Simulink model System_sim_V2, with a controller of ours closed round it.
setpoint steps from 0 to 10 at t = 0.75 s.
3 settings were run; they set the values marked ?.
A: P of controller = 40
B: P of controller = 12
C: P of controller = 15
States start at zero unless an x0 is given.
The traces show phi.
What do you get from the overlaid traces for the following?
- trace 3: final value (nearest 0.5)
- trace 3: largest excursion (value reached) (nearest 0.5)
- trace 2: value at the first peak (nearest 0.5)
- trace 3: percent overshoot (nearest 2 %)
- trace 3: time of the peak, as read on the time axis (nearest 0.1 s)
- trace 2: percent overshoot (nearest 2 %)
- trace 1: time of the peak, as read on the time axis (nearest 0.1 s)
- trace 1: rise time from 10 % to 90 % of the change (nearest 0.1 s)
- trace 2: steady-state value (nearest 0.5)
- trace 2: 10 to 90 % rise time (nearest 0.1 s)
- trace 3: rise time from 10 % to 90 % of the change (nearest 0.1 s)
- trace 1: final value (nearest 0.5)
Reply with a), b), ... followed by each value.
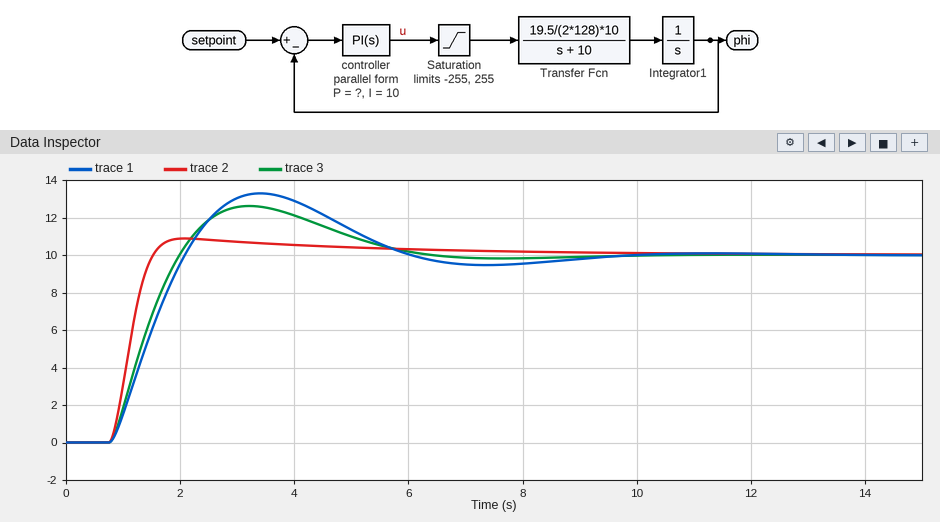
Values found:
a) 10.0
b) 12.5
c) 11.0
d) 26 %
e) 3.2 s
f) 8 %
g) 3.4 s
h) 1.0 s
i) 10.0
j) 0.5 s
k) 0.9 s
l) 10.0
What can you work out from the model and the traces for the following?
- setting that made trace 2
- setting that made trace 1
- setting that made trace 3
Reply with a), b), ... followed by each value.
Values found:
a) A
b) B
c) C
